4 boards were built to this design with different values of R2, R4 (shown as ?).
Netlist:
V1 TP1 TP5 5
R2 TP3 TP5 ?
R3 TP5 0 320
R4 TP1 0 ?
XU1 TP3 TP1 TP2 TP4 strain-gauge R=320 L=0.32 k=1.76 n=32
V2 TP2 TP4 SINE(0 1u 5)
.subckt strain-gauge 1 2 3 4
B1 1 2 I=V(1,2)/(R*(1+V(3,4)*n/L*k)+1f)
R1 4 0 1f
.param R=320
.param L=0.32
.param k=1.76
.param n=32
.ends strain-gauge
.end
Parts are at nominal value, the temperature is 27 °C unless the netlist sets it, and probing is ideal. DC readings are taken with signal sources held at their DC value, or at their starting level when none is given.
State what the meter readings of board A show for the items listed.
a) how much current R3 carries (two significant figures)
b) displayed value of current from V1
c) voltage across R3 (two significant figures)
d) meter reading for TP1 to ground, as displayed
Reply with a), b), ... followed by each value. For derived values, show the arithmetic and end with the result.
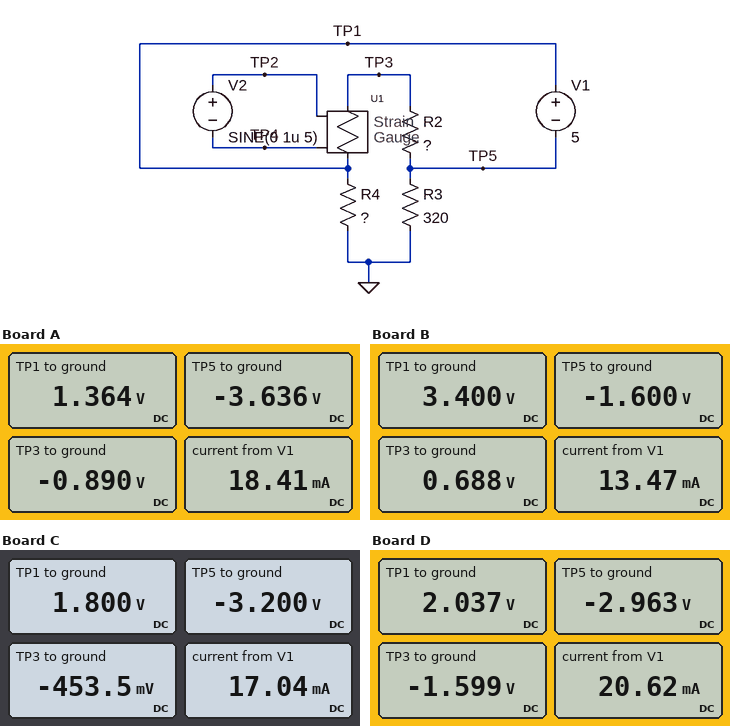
a) (0 V - (-3.636 V)) / 320 Ω = 11 mA
b) 18.41 mA
c) 0 V - (-3.636 V) = 3.6 V
d) 1.364 V
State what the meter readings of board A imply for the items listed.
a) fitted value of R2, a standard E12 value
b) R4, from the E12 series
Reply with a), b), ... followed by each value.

a) 390 Ω
b) 120 Ω
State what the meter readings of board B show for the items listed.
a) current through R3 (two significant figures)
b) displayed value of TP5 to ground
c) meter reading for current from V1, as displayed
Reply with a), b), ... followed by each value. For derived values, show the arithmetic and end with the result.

a) (0 V - (-1.6 V)) / 320 Ω = 5.0 mA
b) -1.600 V
c) 13.47 mA
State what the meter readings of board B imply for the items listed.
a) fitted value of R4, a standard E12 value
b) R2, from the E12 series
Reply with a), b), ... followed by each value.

a) 680 Ω
b) 270 Ω
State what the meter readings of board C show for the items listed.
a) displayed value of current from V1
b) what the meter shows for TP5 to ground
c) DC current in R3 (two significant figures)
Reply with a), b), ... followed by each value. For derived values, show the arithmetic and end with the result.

a) 17.04 mA
b) -3.200 V
c) (0 V - (-3.2 V)) / 320 Ω = 10 mA
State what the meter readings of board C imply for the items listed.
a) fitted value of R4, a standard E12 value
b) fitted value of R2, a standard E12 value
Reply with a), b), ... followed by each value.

a) 180 Ω
b) 390 Ω
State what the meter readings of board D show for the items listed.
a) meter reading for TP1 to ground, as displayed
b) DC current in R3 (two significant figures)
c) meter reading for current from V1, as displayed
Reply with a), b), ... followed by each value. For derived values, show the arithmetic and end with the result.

a) 2.037 V
b) (0 V - (-2.963 V)) / 320 Ω = 9.3 mA
c) 20.62 mA
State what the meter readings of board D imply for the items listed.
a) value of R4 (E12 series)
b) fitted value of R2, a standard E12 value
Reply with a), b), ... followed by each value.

a) 220 Ω
b) 120 Ω
